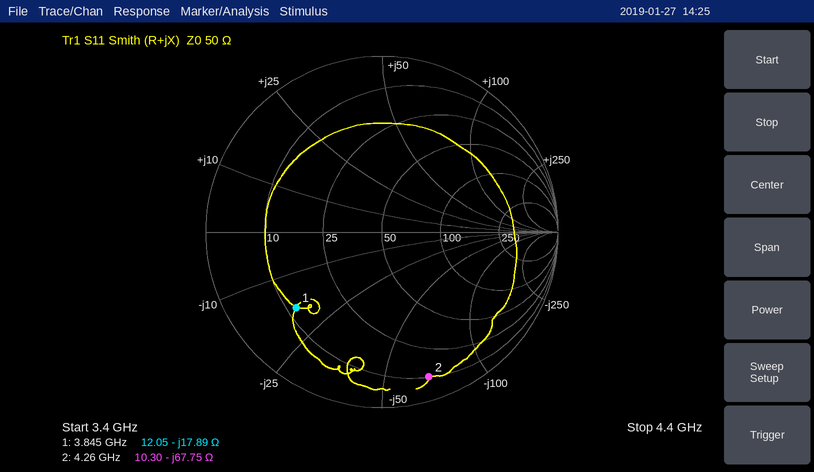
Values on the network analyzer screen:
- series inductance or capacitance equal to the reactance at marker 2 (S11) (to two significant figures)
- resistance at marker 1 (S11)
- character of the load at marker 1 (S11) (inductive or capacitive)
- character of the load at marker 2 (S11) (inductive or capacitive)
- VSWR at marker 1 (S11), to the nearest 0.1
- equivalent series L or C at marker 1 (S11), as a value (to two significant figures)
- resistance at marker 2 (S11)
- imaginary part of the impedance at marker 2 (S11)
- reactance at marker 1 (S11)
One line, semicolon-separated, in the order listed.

550 fF; 12.05 Ω; capacitive; capacitive; 4.7; 2.3 pF; 10.30 Ω; -67.75 Ω; -17.89 Ω
